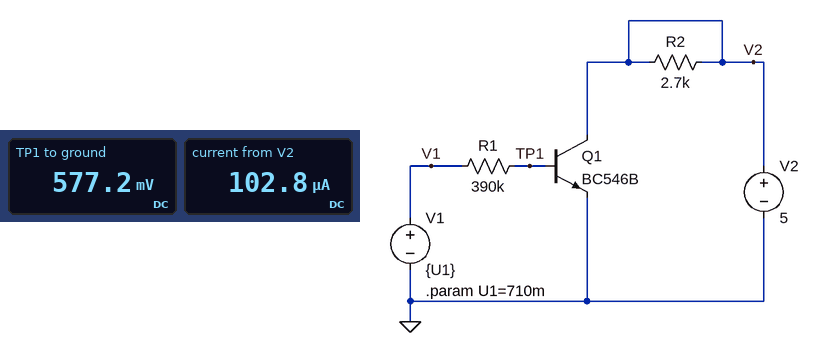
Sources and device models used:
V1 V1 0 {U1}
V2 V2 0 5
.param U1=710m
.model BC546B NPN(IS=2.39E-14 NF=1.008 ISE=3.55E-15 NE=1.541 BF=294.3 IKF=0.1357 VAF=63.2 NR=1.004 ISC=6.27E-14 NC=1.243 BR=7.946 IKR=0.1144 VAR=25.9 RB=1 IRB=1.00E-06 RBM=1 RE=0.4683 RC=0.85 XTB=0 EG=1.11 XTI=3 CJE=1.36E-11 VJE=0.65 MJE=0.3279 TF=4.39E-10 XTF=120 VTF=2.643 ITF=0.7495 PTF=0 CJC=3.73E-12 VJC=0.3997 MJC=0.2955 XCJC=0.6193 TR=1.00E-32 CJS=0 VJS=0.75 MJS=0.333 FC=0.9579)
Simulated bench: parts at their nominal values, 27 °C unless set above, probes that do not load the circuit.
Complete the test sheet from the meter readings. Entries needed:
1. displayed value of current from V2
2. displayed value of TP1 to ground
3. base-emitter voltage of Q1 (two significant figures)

102.8 µA
577.2 mV
580 mV
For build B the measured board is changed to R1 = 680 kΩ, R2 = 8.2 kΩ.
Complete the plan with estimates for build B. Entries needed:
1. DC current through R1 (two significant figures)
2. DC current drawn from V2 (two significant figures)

210 nA
64 µA
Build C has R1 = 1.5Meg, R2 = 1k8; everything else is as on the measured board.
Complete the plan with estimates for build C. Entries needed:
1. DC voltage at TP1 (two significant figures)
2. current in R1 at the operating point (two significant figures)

550 mV
110 nA
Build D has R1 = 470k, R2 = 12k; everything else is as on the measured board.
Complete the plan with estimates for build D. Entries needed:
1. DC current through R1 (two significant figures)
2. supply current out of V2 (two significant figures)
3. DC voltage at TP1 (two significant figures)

290 nA
88 µA
570 mV
